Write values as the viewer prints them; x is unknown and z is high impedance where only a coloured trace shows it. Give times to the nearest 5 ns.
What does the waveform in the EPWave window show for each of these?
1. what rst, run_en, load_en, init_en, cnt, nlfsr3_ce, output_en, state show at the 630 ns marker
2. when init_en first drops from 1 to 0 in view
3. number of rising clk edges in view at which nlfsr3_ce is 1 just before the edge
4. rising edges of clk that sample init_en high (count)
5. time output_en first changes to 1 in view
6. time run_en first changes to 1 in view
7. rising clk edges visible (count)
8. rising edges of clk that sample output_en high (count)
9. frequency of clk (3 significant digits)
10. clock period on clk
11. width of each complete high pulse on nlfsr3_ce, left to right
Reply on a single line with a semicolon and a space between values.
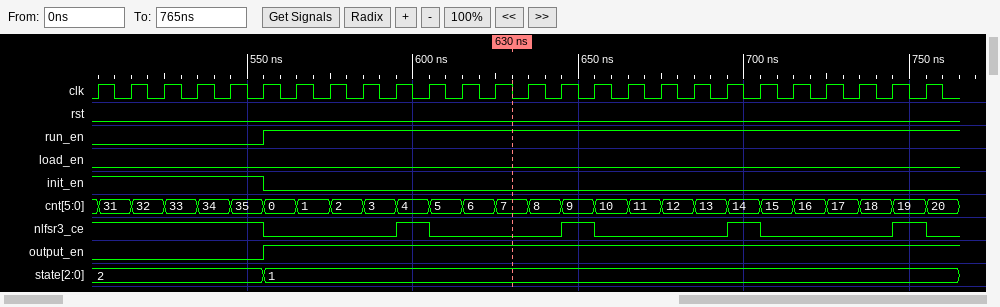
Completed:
rst=0, run_en=1, load_en=0, init_en=0, cnt=7, nlfsr3_ce=0, output_en=1, state=1; 555 ns; 10; 6; 555 ns; 555 ns; 26; 20; 100 MHz; 10 ns; 10 ns, 10 ns, 10 ns, 10 ns
